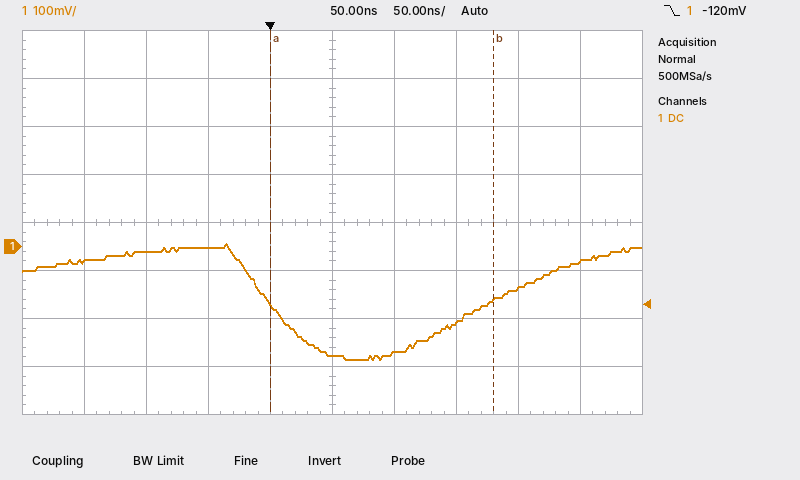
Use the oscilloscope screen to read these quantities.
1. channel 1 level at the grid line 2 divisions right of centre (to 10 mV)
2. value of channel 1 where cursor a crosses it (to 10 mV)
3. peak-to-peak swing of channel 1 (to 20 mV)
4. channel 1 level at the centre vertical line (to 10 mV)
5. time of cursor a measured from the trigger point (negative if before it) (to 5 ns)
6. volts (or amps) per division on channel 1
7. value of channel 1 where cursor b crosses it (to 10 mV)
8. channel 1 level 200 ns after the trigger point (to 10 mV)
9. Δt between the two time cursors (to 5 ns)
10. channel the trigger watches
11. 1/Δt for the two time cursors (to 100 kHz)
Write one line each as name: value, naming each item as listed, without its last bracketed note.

channel 1 level at the grid line 2 divisions right of centre: -160 mV
value of channel 1 where cursor a crosses it: -120 mV
peak-to-peak swing of channel 1: 240 mV
channel 1 level at the centre vertical line: -230 mV
time of cursor a measured from the trigger point (negative if before it): 0 ns
volts (or amps) per division on channel 1: 100 mV
value of channel 1 where cursor b crosses it: -110 mV
channel 1 level 200 ns after the trigger point: -90 mV
Δt between the two time cursors: 180 ns
channel the trigger watches: channel 1
1/Δt for the two time cursors: 5.6 MHz
